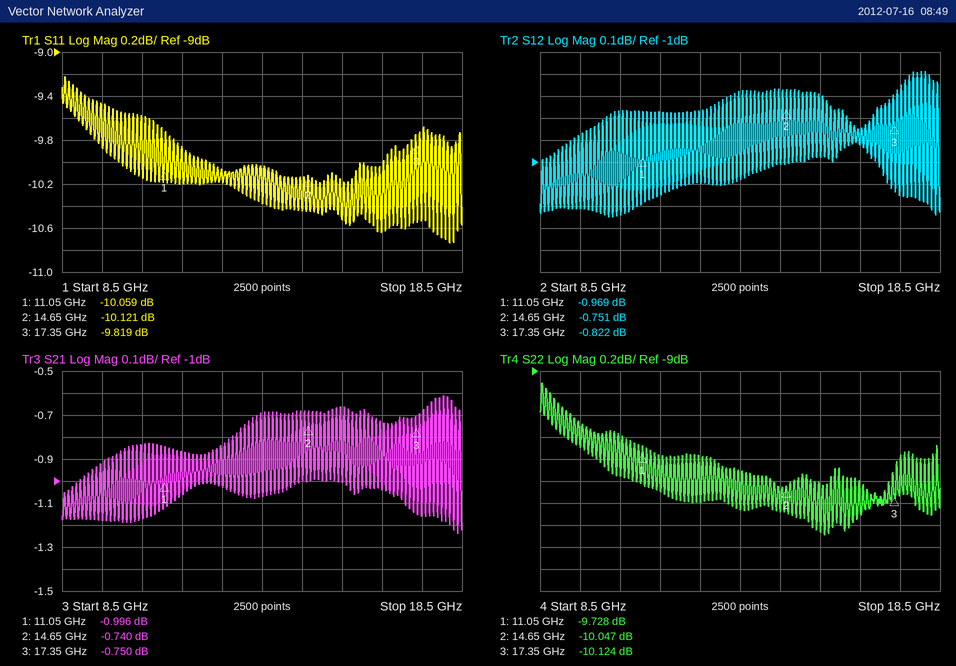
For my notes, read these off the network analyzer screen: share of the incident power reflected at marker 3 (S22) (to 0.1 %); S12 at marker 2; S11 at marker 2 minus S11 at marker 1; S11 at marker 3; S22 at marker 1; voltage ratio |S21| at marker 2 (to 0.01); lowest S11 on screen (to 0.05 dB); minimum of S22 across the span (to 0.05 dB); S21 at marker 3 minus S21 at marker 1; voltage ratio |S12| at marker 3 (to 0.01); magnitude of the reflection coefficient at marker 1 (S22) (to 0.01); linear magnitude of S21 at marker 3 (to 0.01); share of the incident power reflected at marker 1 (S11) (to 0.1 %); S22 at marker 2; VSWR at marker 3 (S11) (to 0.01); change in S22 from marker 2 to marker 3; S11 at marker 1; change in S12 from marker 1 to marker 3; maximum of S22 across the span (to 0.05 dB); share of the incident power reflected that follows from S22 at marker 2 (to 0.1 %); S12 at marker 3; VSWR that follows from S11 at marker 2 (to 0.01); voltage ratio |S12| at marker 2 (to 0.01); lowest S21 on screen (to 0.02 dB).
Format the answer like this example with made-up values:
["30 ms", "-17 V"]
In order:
["9.7 %", "-0.751 dB", "-0.062 dB", "-9.819 dB", "-9.728 dB", "0.92", "-10.75 dB", "-10.50 dB", "0.246 dB", "0.91", "0.33", "0.92", "9.9 %", "-10.047 dB", "1.95", "-0.077 dB", "-10.059 dB", "0.147 dB", "-9.10 dB", "9.9 %", "-0.822 dB", "1.91", "0.92", "-1.24 dB"]
